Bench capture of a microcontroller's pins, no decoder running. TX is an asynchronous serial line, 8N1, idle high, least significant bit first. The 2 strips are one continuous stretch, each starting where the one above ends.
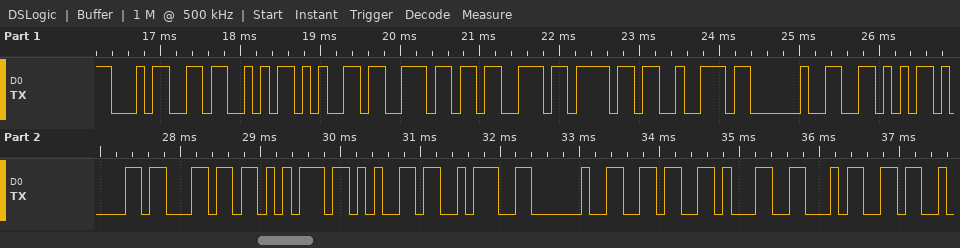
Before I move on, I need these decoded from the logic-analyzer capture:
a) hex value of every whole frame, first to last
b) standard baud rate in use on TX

34 53 65 6E 73 6F 72 20 56 61 6C 75 65 3A 20 36 31 34
9600 baud
